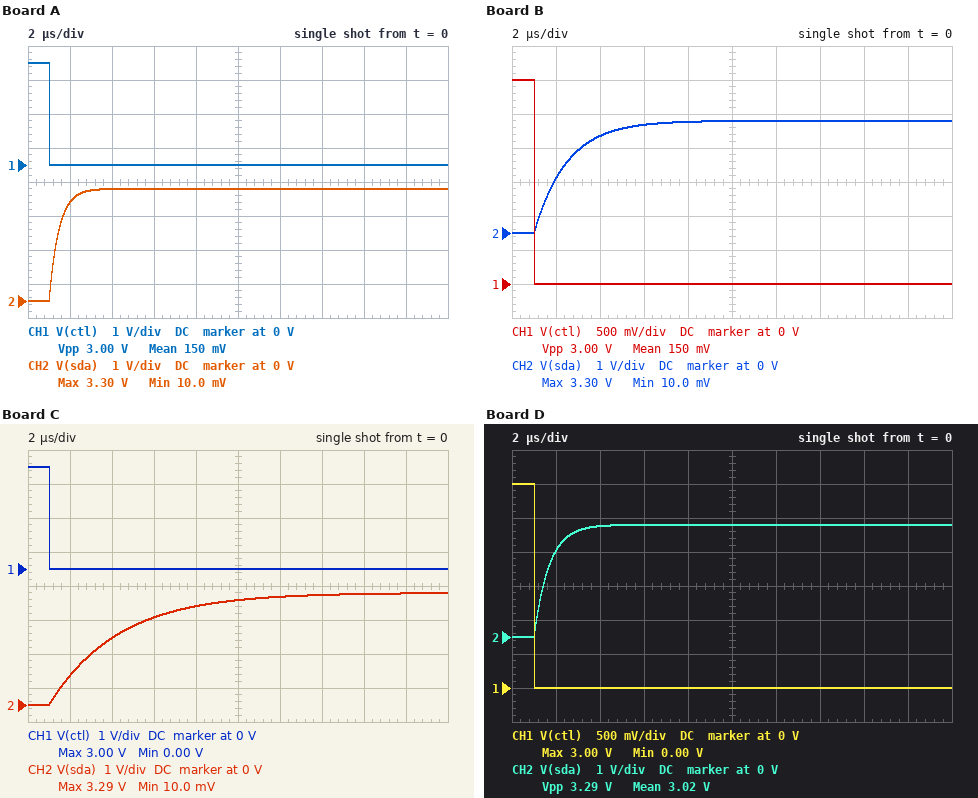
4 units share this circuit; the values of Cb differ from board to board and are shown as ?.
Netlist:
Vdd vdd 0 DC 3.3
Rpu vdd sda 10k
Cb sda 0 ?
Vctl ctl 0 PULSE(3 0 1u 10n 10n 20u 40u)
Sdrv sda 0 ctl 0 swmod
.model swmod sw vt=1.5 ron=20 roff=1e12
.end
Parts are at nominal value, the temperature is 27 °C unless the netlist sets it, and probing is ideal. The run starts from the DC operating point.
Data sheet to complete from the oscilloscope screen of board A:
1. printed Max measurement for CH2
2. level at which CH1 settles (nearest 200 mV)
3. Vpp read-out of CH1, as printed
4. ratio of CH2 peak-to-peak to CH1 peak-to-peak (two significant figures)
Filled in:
3.30 V
0 V
3.00 V
1.1
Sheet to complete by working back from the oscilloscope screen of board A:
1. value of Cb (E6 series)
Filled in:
47 pF
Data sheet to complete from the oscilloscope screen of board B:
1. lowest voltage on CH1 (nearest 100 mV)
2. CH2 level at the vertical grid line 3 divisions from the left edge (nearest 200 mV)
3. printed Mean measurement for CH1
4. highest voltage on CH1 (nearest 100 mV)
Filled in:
0 V
3.2 V
150 mV
3.0 V
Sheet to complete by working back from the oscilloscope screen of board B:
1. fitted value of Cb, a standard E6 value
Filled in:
150 pF
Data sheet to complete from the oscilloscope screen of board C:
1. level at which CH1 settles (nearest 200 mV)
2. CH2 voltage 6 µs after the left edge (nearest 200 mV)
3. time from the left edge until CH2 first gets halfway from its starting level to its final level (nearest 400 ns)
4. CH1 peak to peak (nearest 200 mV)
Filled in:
0 V
2.6 V
3.2 µs
3.0 V
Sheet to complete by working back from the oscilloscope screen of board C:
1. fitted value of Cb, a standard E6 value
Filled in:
330 pF
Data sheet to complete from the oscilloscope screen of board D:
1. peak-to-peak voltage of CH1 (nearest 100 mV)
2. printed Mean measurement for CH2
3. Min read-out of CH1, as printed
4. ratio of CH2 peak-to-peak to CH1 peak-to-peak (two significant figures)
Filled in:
3.0 V
3.02 V
0.00 V
1.1
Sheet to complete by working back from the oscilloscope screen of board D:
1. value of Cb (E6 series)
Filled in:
68 pF
